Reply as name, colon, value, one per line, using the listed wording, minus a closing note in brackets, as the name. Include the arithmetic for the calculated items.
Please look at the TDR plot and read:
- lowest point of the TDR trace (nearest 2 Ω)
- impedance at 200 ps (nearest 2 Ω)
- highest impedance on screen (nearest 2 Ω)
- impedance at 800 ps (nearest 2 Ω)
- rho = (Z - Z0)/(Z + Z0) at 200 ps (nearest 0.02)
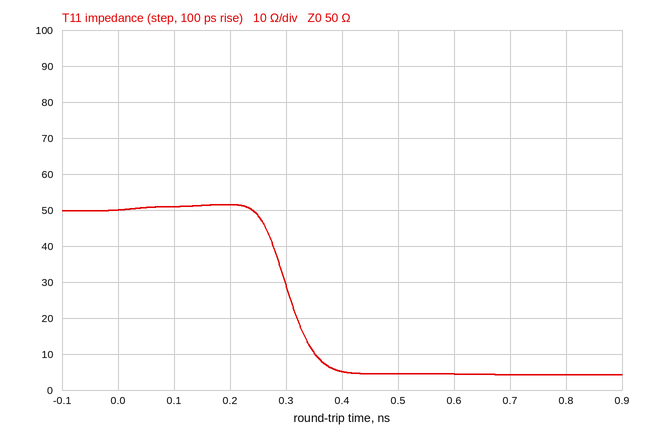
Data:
lowest point of the TDR trace: 4 Ω
impedance at 200 ps: 52 Ω
highest impedance on screen: 52 Ω
impedance at 800 ps: 4 Ω
rho = (Z - Z0)/(Z + Z0) at 200 ps: (52 − 50)/(52 + 50) ≈ +0.02
